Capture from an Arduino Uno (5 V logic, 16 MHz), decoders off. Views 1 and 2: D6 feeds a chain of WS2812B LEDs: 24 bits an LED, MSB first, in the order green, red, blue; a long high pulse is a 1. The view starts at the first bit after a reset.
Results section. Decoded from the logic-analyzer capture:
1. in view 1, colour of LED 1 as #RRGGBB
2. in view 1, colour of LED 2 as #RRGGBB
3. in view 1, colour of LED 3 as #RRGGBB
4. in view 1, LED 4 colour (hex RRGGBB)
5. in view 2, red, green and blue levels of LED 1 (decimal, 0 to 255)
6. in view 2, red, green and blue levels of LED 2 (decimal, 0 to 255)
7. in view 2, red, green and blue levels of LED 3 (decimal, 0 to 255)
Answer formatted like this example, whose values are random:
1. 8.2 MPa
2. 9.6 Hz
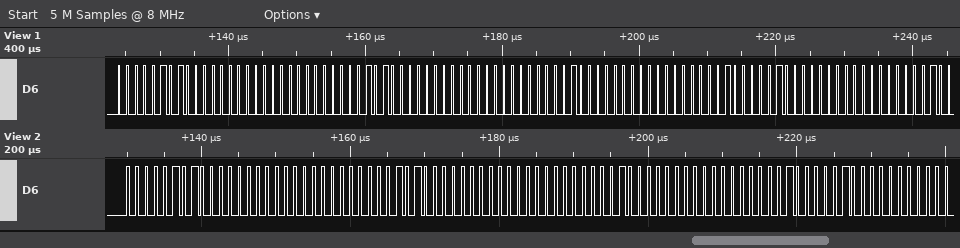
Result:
1. #000500
2. #000500
3. #000401
4. #000401
5. 0, 5, 0
6. 0, 5, 0
7. 0, 4, 1
